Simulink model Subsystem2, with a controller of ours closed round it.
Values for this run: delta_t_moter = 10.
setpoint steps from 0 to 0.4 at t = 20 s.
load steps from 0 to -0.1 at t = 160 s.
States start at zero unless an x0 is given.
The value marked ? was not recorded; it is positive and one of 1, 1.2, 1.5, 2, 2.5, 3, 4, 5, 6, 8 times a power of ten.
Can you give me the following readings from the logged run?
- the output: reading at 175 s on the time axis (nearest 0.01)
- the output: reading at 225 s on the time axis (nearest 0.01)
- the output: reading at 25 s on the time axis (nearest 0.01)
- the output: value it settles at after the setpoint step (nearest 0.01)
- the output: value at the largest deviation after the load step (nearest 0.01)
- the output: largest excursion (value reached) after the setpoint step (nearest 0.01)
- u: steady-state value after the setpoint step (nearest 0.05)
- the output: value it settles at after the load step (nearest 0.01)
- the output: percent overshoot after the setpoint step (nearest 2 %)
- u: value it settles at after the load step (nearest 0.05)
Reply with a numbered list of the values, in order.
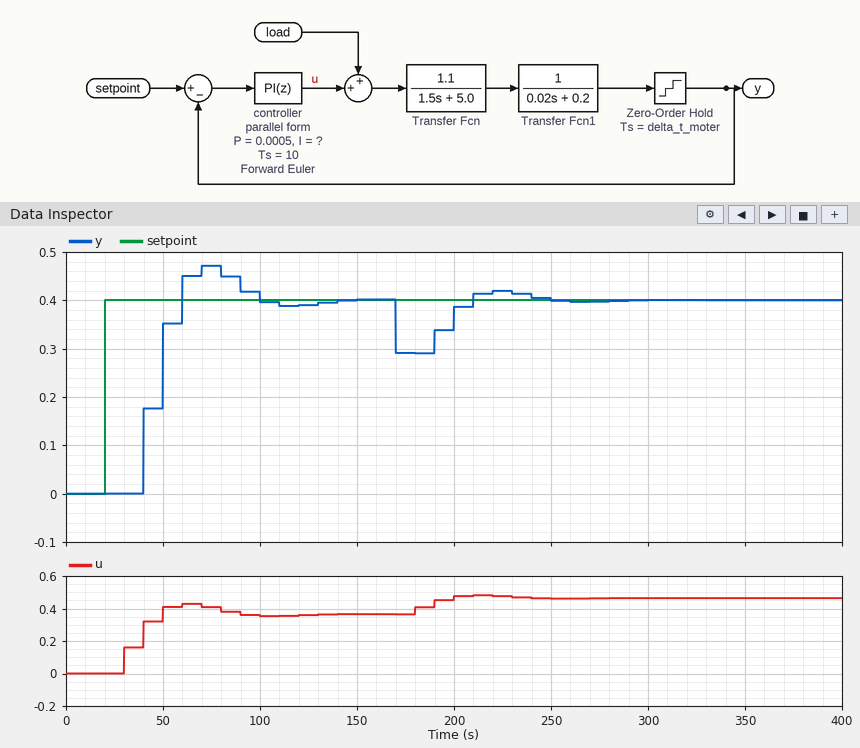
1. 0.29
2. 0.42
3. 0.00
4. 0.40
5. 0.29
6. 0.47
7. 0.35
8. 0.40
9. 18 %
10. 0.45
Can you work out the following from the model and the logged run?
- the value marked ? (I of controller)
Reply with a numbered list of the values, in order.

1. 0.04
